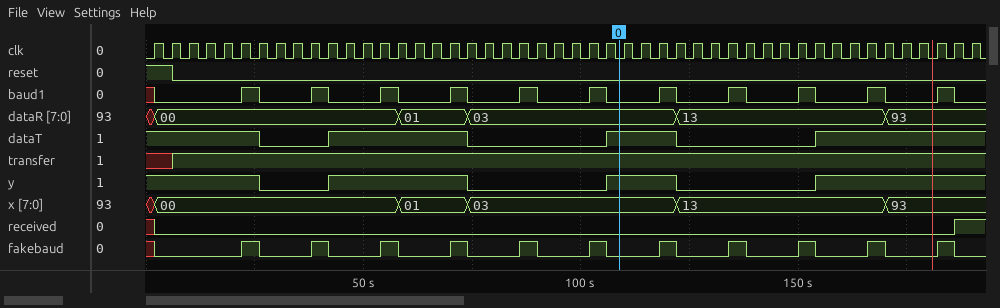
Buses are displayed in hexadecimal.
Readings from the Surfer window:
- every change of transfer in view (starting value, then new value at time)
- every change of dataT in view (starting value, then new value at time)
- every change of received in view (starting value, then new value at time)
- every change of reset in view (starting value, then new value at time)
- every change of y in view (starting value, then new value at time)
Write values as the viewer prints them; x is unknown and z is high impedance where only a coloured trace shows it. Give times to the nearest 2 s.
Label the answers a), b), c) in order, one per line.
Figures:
a) x, 1 at 6 s
b) 1, 0 at 26 s, 1 at 42 s, 0 at 74 s, 1 at 106 s, 0 at 122 s, 1 at 154 s
c) x, 0 at 2 s, 1 at 186 s
d) 1, 0 at 6 s
e) 1, 0 at 26 s, 1 at 42 s, 0 at 74 s, 1 at 106 s, 0 at 122 s, 1 at 154 s
